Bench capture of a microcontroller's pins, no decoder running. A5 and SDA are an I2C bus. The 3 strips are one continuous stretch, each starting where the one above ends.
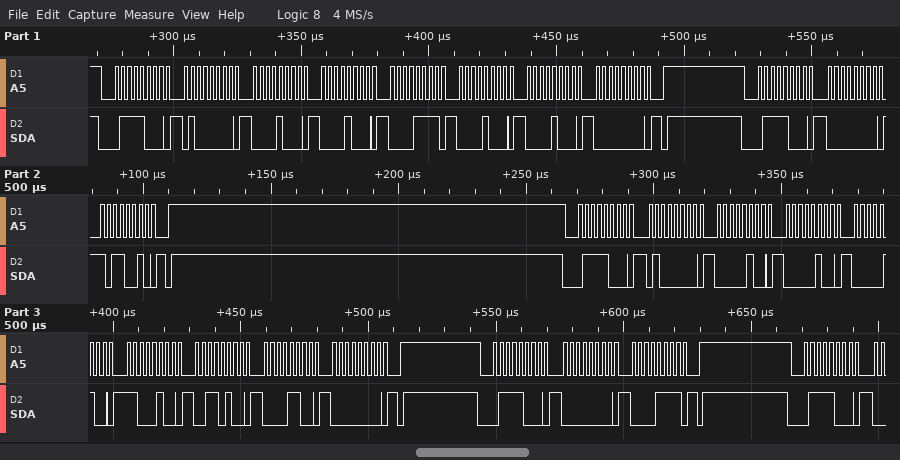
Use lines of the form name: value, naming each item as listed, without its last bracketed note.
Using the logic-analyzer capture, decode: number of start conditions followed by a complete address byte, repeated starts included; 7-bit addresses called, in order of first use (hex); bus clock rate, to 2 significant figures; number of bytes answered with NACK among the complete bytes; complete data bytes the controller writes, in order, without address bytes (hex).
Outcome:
number of start conditions followed by a complete address byte, repeated starts included: 5
7-bit addresses called, in order of first use: 0x3C
bus clock rate, to 2 significant figures: 400 kHz
number of bytes answered with NACK among the complete bytes: 0
complete data bytes the controller writes, in order, without address bytes: 40 08 08 0F 08 08 00 00 B2 40 04 04 04 C4 34 0C 00 00 0F
